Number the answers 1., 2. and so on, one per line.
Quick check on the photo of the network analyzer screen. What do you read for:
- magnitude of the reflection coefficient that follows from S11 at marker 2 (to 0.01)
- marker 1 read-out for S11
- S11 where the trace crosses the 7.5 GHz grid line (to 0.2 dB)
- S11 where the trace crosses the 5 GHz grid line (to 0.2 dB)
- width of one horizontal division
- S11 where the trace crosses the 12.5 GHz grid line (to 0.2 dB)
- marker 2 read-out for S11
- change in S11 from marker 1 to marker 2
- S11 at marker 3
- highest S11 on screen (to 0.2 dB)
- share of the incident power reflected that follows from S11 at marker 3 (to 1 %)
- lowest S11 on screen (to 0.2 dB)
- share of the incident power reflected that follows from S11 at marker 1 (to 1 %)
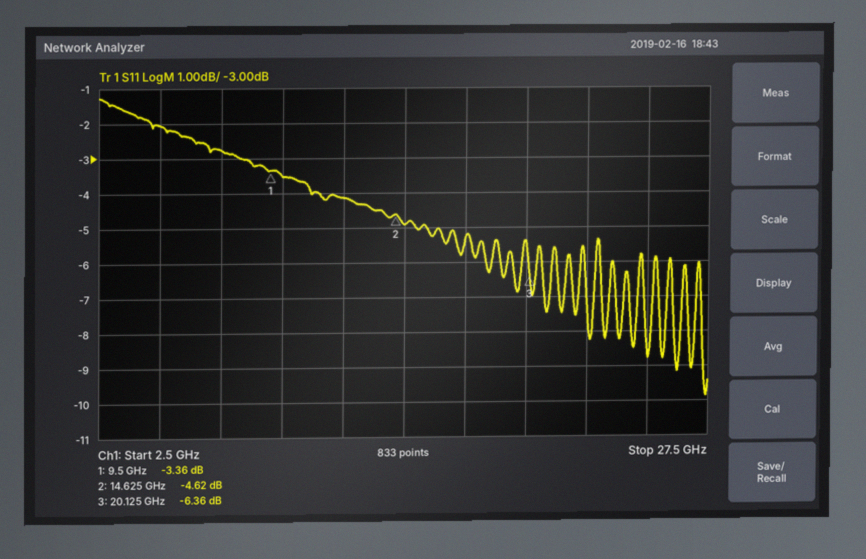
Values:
1. 0.59
2. -3.36 dB
3. -2.8 dB
4. -2.0 dB
5. 2.5 GHz
6. -4.2 dB
7. -4.62 dB
8. -1.26 dB
9. -6.36 dB
10. -1.2 dB
11. 23 %
12. -9.8 dB
13. 46 %
